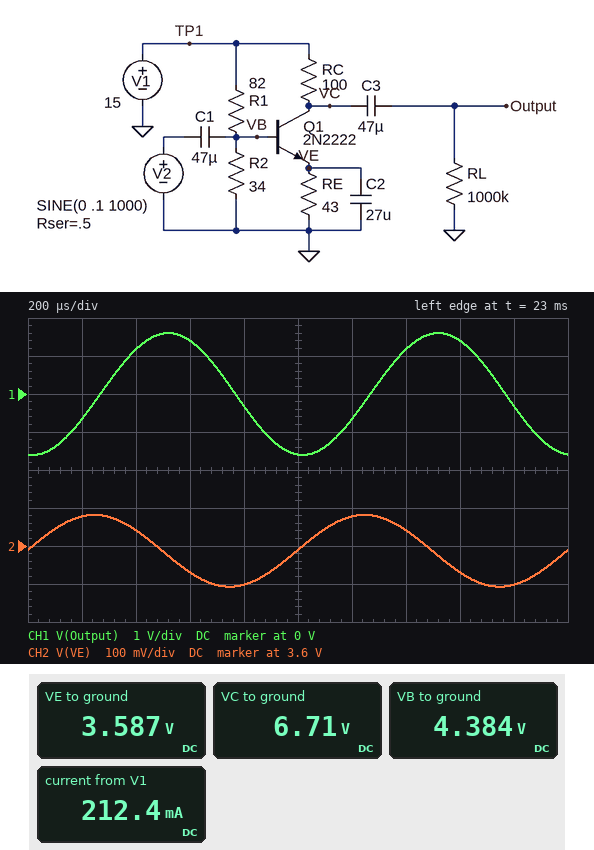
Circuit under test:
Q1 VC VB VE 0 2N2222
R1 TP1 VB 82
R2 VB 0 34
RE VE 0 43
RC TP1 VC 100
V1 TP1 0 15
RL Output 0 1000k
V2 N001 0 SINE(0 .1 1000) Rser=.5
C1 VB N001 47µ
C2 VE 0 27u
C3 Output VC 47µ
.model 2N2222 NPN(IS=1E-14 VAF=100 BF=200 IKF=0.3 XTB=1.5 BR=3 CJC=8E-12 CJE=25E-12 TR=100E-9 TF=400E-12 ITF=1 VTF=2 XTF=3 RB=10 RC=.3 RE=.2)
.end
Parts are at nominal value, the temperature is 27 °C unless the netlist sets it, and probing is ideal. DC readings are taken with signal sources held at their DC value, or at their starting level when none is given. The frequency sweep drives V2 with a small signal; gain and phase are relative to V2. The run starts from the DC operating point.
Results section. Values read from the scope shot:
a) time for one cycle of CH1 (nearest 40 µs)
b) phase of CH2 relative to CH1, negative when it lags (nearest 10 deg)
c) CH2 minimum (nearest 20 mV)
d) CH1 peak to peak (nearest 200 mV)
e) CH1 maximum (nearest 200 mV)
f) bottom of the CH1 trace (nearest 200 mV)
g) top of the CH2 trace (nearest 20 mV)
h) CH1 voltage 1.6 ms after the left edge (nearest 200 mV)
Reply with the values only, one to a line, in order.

1.00 ms
100 deg
3.50 V
3.2 V
1.6 V
-1.6 V
3.68 V
1.4 V
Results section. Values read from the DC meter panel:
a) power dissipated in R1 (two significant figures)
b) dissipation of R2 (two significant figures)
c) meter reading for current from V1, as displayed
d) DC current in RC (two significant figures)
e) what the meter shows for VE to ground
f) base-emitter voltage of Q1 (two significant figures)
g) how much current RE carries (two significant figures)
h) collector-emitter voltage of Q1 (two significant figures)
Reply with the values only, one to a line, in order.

1.4 W
570 mW
212.4 mA
83 mA
3.587 V
800 mV
83 mA
3.1 V
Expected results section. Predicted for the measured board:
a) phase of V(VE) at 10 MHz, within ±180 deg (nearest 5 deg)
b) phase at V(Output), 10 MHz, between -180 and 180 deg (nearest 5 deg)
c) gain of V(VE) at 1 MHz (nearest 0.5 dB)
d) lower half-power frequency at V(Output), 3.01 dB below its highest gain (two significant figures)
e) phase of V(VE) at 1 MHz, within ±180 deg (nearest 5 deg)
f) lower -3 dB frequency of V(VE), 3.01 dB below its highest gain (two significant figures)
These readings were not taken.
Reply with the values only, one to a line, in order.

-130 deg
135 deg
-41.5 dB
8.7 kHz
-95 deg
130 Hz
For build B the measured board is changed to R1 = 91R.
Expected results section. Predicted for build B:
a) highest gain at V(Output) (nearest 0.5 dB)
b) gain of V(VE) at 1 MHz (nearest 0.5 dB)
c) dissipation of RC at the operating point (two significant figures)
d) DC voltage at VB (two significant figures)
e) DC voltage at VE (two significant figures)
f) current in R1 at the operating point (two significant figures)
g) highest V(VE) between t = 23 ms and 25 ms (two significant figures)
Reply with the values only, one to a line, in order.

42.5 dB
-42.0 dB
570 mW
4.1 V
3.3 V
120 mA
3.4 V
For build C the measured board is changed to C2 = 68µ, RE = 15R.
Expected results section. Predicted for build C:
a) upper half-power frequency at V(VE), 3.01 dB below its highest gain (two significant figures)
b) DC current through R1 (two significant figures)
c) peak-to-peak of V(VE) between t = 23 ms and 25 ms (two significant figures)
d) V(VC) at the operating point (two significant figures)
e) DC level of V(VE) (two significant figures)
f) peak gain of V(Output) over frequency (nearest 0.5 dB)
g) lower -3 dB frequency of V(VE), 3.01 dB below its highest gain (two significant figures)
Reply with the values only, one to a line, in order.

930 Hz
140 mA
34 mV
2.5 V
2.4 V
-12.0 dB
110 Hz
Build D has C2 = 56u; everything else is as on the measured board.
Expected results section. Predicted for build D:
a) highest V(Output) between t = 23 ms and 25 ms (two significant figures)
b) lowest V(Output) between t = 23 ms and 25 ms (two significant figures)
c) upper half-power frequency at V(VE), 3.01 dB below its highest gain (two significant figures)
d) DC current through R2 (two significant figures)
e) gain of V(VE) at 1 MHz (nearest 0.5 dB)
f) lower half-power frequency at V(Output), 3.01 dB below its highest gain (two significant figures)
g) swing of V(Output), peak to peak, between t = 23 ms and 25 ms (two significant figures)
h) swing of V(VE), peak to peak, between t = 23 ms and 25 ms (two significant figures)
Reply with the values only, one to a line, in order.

3.2 V
-2.9 V
4.5 kHz
130 mA
-48.0 dB
4.2 kHz
6.1 V
180 mV
